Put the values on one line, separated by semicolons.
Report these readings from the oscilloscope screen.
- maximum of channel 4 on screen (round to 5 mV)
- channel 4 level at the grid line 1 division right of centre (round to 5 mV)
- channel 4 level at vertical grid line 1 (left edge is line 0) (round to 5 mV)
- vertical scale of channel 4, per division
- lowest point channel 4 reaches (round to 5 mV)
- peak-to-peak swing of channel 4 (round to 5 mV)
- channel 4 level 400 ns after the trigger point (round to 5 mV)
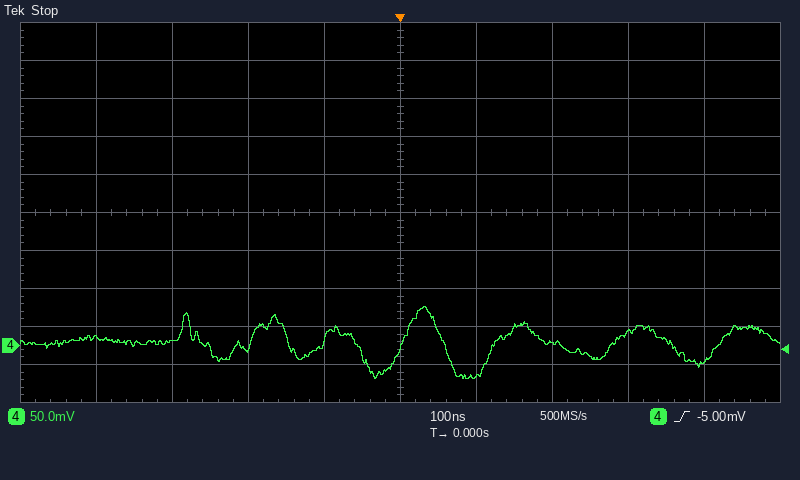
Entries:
50 mV; -40 mV; 10 mV; 50 mV; -45 mV; 95 mV; -20 mV
